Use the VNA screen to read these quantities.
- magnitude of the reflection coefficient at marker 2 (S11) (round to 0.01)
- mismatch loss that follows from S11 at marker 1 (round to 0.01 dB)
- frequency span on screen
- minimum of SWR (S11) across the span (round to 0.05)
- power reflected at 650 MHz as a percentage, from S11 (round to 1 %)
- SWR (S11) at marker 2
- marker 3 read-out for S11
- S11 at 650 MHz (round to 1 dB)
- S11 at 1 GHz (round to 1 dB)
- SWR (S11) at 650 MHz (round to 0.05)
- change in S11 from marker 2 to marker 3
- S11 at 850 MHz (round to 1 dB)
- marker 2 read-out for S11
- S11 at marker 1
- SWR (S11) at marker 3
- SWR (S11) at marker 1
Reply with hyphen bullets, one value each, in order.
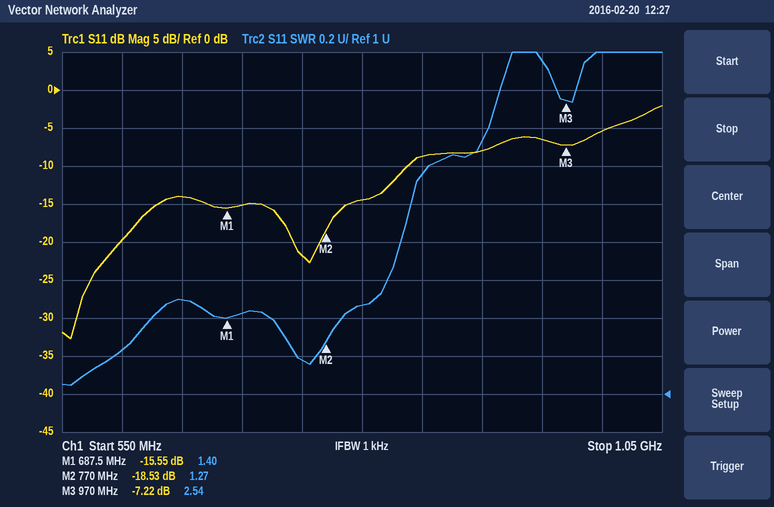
- 0.12
- 0.12 dB
- 500 MHz
- 1.05
- 4 %
- 1.27
- -7.22 dB
- -14 dB
- -5 dB
- 1.50
- 11.31 dB
- -9 dB
- -18.53 dB
- -15.55 dB
- 2.54
- 1.40
